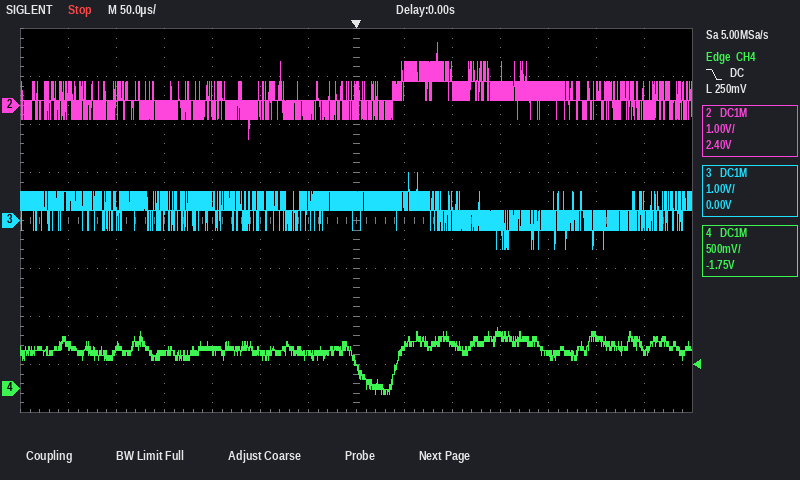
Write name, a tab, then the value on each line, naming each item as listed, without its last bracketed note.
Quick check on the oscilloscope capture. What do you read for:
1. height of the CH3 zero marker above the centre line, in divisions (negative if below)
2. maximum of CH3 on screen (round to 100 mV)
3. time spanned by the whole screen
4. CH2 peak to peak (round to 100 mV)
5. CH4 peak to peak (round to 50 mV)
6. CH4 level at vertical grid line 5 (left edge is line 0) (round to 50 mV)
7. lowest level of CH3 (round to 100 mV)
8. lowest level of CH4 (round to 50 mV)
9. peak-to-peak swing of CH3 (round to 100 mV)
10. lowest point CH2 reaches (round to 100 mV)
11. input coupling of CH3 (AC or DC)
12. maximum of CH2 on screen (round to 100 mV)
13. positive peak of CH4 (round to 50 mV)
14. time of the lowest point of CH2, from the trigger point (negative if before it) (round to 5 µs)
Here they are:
height of the CH3 zero marker above the centre line, in divisions	0.0 div
maximum of CH3 on screen	1.0 V
time spanned by the whole screen	700 µs
CH2 peak to peak	2.0 V
CH4 peak to peak	700 mV
CH4 level at vertical grid line 5 (left edge is line 0)	400 mV
lowest level of CH3	-600 mV
lowest level of CH4	-50 mV
peak-to-peak swing of CH3	1.6 V
lowest point CH2 reaches	-700 mV
input coupling of CH3	DC
maximum of CH2 on screen	1.3 V
positive peak of CH4	650 mV
time of the lowest point of CH2, from the trigger point (negative if before it)	-110 µs
